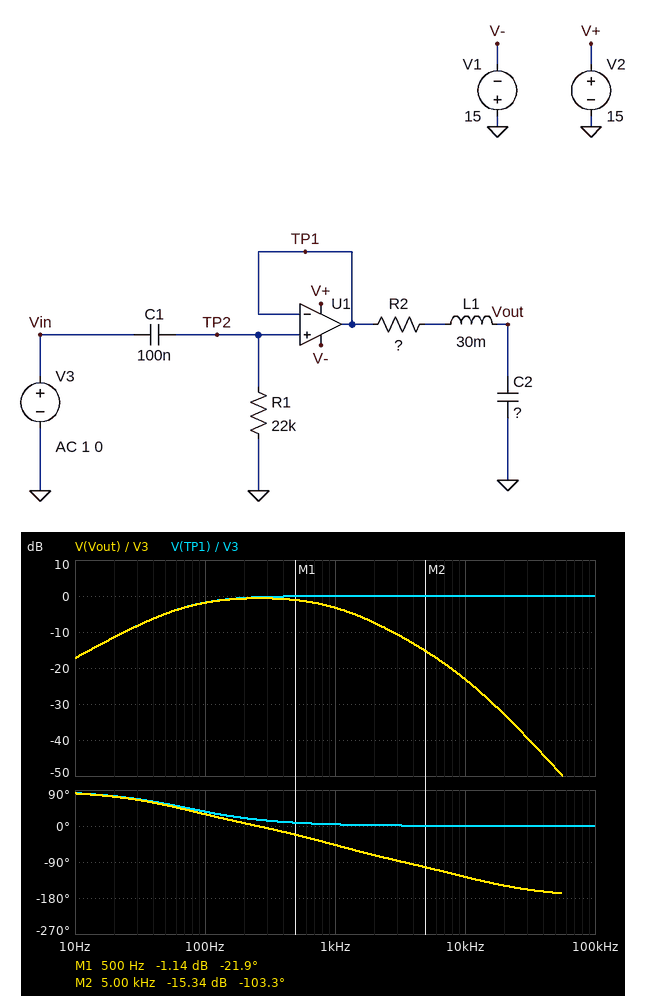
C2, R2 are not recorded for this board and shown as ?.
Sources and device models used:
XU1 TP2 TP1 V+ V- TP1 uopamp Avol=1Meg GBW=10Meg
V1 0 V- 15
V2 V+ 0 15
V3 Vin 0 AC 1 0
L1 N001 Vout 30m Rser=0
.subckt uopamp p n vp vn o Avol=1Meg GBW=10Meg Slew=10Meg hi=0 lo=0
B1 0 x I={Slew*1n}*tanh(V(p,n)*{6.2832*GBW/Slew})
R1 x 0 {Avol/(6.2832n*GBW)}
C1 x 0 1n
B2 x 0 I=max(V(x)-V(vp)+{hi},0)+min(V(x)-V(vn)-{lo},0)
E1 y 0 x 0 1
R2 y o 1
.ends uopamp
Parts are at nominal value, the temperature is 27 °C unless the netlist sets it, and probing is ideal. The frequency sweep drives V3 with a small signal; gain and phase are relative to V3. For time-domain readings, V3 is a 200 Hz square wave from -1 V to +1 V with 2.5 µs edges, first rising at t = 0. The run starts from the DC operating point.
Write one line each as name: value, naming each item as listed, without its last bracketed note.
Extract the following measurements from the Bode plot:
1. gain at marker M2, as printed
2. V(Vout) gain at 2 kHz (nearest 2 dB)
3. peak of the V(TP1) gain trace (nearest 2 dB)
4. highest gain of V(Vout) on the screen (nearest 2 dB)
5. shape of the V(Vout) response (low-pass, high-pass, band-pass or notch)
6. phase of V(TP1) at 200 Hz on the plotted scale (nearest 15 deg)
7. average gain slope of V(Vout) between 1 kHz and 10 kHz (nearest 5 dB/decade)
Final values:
gain at marker M2, as printed: -15.34 dB
V(Vout) gain at 2 kHz: -8 dB
peak of the V(TP1) gain trace: 0 dB
highest gain of V(Vout) on the screen: 0 dB
shape of the V(Vout) response: band-pass
phase of V(TP1) at 200 Hz on the plotted scale: 15 deg
average gain slope of V(Vout) between 1 kHz and 10 kHz: -20 dB/decade
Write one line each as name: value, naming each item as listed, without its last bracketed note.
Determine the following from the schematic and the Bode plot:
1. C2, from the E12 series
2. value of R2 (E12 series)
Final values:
C2, from the E12 series: 82 nF
value of R2: 2.2 kΩ
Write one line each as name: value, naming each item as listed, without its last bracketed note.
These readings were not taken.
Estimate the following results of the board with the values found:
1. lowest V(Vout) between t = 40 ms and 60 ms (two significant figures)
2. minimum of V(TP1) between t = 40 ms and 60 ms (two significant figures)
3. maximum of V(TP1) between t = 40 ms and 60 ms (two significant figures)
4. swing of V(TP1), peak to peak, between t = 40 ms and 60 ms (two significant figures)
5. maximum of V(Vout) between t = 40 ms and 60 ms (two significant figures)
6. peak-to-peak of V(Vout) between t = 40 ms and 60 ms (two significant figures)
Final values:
lowest V(Vout) between t = 40 ms and 60 ms: -1.2 V
minimum of V(TP1) between t = 40 ms and 60 ms: -1.5 V
maximum of V(TP1) between t = 40 ms and 60 ms: 1.5 V
swing of V(TP1), peak to peak, between t = 40 ms and 60 ms: 3.0 V
maximum of V(Vout) between t = 40 ms and 60 ms: 1.2 V
peak-to-peak of V(Vout) between t = 40 ms and 60 ms: 2.4 V
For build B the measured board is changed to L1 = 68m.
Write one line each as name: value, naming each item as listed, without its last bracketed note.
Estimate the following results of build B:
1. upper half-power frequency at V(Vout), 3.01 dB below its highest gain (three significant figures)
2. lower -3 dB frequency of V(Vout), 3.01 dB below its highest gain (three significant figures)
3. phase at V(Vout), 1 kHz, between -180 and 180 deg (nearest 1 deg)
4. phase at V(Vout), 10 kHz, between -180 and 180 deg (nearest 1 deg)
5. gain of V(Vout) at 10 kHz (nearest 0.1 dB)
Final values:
upper half-power frequency at V(Vout), 3.01 dB below its highest gain: 1.18 kHz
lower -3 dB frequency of V(Vout), 3.01 dB below its highest gain: 64.3 Hz
phase at V(Vout), 1 kHz, between -180 and 180 deg: -51 deg
phase at V(Vout), 10 kHz, between -180 and 180 deg: -151 deg
gain of V(Vout) at 10 kHz: -27.6 dB
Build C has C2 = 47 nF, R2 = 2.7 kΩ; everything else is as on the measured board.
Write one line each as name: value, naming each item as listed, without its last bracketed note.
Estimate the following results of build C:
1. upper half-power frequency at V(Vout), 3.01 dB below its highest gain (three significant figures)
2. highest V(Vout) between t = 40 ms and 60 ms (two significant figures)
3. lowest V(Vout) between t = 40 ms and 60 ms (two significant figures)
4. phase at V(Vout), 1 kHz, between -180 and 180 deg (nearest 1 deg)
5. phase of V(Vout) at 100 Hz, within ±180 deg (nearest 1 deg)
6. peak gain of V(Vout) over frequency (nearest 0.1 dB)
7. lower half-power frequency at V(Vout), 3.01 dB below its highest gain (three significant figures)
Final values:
upper half-power frequency at V(Vout), 3.01 dB below its highest gain: 1.51 kHz
highest V(Vout) between t = 40 ms and 60 ms: 1.3 V
lowest V(Vout) between t = 40 ms and 60 ms: -1.3 V
phase at V(Vout), 1 kHz, between -180 and 180 deg: -36 deg
phase of V(Vout) at 100 Hz, within ±180 deg: 31 deg
peak gain of V(Vout) over frequency: -0.4 dB
lower half-power frequency at V(Vout), 3.01 dB below its highest gain: 65.8 Hz
